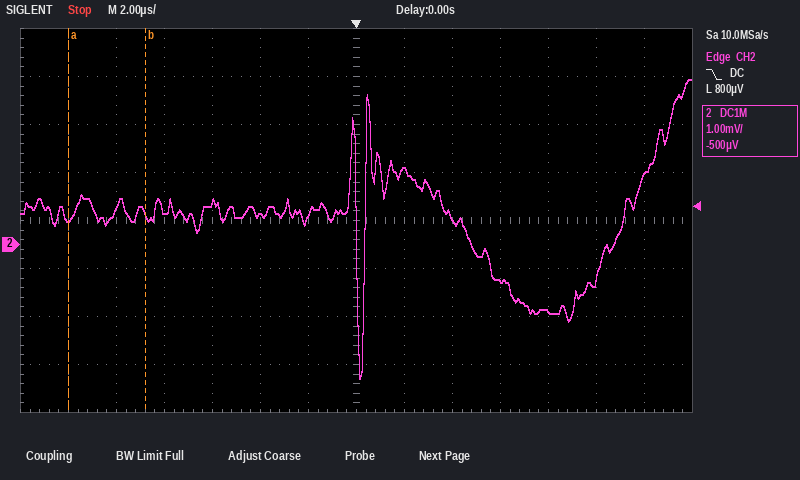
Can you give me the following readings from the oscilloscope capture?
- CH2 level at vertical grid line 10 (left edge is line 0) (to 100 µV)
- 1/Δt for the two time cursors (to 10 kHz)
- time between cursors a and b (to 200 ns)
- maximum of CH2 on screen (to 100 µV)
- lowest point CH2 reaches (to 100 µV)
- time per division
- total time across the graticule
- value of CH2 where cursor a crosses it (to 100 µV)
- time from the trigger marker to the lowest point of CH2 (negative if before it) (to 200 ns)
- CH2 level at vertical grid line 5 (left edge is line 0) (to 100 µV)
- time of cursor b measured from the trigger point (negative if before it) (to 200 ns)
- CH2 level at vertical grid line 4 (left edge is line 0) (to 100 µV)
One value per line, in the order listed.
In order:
-800 µV
310 kHz
3.2 µs
3.4 mV
-2.8 mV
2 µs
28 µs
500 µV
+200 ns
600 µV
-8.8 µs
900 µV
